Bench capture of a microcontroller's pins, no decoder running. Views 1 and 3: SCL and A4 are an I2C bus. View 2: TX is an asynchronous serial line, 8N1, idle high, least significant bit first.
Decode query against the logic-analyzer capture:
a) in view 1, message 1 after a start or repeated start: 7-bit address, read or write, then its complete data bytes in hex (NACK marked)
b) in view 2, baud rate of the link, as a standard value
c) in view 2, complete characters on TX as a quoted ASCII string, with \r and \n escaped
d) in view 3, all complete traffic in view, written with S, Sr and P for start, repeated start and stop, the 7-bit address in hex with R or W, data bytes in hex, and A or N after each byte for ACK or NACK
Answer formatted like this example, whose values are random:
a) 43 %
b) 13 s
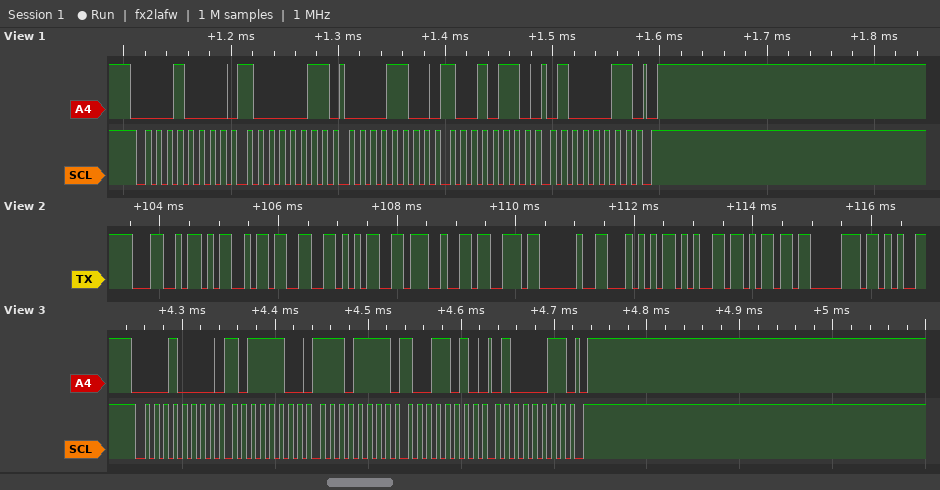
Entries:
a) 0x08 write: 83 0C 96 43
b) 9600 baud
c) "LM35's Temp"
d) S 08W A BC A EF A 9A A 43 A P
